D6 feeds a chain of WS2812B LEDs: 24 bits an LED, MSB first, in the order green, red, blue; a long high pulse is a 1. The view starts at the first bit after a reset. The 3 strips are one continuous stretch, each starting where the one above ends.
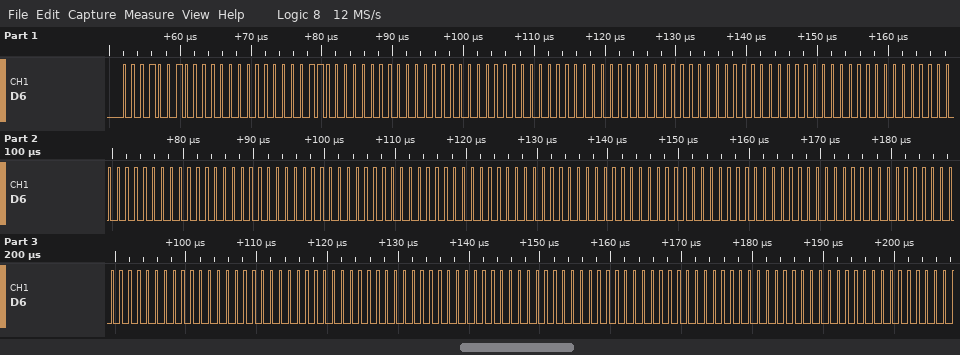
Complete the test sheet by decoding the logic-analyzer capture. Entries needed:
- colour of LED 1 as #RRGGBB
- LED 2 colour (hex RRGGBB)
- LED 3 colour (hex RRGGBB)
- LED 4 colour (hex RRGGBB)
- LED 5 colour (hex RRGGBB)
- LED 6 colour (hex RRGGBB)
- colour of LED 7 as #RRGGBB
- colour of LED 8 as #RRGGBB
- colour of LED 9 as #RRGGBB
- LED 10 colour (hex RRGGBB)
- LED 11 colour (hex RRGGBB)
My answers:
#001206
#000000
#000000
#000000
#000000
#000000
#000000
#000000
#000000
#000000
#000000
